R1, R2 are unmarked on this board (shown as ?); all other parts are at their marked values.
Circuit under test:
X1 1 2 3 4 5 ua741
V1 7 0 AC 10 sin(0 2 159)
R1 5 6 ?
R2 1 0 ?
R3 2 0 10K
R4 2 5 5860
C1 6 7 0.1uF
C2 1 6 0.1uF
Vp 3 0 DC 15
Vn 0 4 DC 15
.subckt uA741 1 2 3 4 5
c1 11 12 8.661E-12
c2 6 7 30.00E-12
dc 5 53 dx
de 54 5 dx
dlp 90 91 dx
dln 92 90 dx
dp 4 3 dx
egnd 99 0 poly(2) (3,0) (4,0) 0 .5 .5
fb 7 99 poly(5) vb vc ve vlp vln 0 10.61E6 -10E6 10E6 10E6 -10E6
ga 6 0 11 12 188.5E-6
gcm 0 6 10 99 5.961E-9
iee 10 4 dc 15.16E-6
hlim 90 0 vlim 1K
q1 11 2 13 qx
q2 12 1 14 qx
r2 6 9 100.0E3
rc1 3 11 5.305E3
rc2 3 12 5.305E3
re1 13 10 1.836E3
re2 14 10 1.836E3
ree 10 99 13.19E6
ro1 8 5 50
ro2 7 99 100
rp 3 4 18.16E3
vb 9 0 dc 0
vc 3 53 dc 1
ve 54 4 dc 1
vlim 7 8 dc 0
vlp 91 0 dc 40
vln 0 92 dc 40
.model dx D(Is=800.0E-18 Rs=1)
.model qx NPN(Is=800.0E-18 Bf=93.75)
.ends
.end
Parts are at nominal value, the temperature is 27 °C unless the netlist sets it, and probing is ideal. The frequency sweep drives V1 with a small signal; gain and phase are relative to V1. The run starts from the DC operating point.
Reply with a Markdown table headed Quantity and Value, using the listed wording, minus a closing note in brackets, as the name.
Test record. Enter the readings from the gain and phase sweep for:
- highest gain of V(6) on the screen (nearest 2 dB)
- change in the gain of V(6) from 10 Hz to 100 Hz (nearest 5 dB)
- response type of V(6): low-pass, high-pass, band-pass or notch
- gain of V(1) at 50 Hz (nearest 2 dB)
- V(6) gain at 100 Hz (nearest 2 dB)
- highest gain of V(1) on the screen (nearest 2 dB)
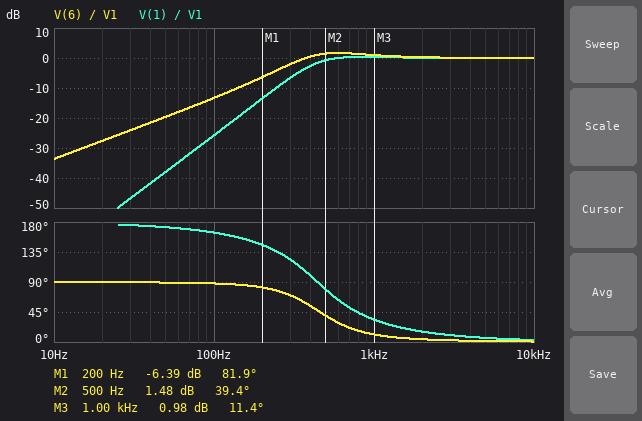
| Quantity | Value |
|---|---|
| highest gain of V(6) on the screen | 2 dB |
| change in the gain of V(6) from 10 Hz to 100 Hz | 20 dB |
| response type of V(6): low-pass, high-pass, band-pass or notch | high-pass |
| gain of V(1) at 50 Hz | -38 dB |
| V(6) gain at 100 Hz | -14 dB |
| highest gain of V(1) on the screen | 0 dB |
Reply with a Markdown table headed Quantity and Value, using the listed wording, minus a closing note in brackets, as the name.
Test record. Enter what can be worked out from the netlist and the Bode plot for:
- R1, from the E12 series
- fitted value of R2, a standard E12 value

| Quantity | Value |
|---|---|
| R1, from the E12 series | 3.3 kΩ |
| fitted value of R2, a standard E12 value | 3.9 kΩ |
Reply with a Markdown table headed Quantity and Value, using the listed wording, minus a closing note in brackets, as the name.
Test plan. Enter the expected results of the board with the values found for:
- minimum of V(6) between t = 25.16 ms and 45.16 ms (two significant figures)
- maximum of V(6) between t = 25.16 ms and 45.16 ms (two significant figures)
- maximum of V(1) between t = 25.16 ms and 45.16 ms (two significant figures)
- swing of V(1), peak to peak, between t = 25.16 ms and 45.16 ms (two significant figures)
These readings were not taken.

| Quantity | Value |
|---|---|
| minimum of V(6) between t = 25.16 ms and 45.16 ms | -730 mV |
| maximum of V(6) between t = 25.16 ms and 45.16 ms | 730 mV |
| maximum of V(1) between t = 25.16 ms and 45.16 ms | 260 mV |
| swing of V(1), peak to peak, between t = 25.16 ms and 45.16 ms | 530 mV |
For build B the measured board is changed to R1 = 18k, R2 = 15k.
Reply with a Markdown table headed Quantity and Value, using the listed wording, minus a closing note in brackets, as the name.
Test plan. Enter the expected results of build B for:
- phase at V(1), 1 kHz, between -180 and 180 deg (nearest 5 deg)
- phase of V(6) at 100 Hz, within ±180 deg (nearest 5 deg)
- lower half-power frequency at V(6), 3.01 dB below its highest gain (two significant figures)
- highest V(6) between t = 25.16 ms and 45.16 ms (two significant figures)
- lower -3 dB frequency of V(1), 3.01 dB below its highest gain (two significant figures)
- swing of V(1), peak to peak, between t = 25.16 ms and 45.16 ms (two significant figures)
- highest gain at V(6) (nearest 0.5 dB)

| Quantity | Value |
|---|---|
| phase at V(1), 1 kHz, between -180 and 180 deg | 10 deg |
| phase of V(6) at 100 Hz, within ±180 deg | 40 deg |
| lower half-power frequency at V(6), 3.01 dB below its highest gain | 68 Hz |
| highest V(6) between t = 25.16 ms and 45.16 ms | 2.0 V |
| lower -3 dB frequency of V(1), 3.01 dB below its highest gain | 120 Hz |
| swing of V(1), peak to peak, between t = 25.16 ms and 45.16 ms | 3.4 V |
| highest gain at V(6) | 0 dB |
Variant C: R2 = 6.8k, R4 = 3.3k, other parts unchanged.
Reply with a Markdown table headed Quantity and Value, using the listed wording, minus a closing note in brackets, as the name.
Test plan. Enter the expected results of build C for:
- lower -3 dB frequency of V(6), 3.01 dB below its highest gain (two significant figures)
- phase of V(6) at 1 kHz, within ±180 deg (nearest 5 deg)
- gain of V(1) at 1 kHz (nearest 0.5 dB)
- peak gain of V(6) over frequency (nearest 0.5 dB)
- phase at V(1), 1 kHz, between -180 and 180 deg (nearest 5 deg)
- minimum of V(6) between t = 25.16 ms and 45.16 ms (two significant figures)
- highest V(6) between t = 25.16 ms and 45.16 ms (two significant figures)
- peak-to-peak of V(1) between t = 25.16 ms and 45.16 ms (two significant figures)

| Quantity | Value |
|---|---|
| lower -3 dB frequency of V(6), 3.01 dB below its highest gain | 260 Hz |
| phase of V(6) at 1 kHz, within ±180 deg | 5 deg |
| gain of V(1) at 1 kHz | 0.5 dB |
| peak gain of V(6) over frequency | 3.0 dB |
| phase at V(1), 1 kHz, between -180 and 180 deg | 20 deg |
| minimum of V(6) between t = 25.16 ms and 45.16 ms | -900 mV |
| highest V(6) between t = 25.16 ms and 45.16 ms | 900 mV |
| peak-to-peak of V(1) between t = 25.16 ms and 45.16 ms | 1.0 V |
